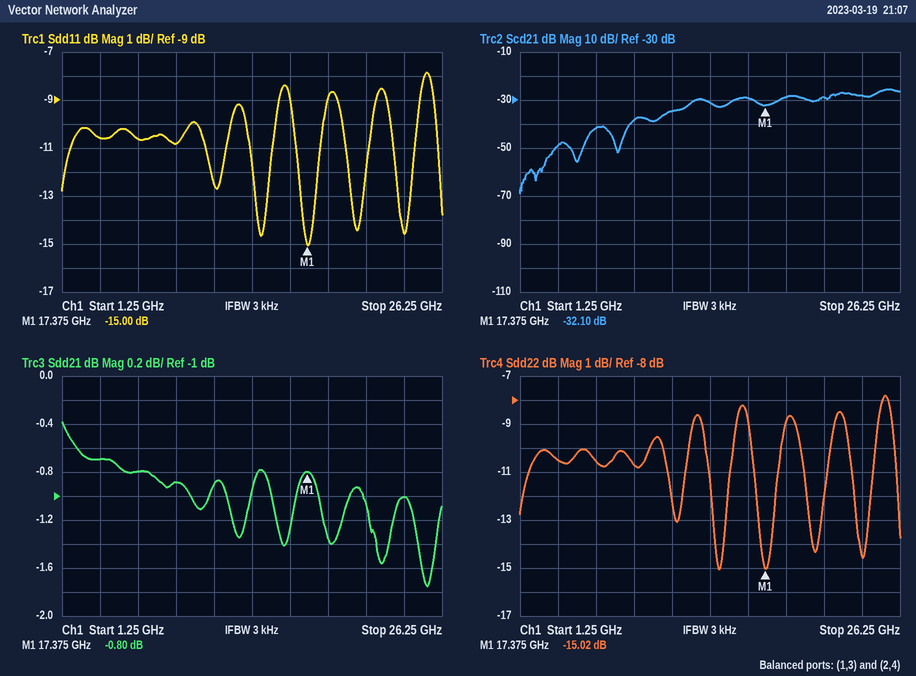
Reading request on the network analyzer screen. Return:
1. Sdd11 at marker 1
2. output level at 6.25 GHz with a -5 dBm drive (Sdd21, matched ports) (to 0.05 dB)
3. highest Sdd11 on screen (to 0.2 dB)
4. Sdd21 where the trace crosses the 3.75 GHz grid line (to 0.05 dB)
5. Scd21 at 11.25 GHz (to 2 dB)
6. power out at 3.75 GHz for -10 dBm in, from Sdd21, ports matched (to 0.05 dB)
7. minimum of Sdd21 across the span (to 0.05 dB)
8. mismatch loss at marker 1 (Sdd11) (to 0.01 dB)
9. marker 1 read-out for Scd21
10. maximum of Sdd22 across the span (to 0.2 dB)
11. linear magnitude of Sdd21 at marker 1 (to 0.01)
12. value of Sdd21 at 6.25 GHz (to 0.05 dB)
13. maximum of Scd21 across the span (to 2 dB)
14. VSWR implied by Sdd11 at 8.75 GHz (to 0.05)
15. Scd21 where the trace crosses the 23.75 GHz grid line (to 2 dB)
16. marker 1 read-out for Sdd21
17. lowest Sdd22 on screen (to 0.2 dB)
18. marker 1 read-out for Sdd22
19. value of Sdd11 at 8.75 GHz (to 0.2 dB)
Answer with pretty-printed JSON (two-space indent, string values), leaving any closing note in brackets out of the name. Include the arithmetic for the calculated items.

{
  "Sdd11 at marker 1": "-15.00 dB",
  "output level at 6.25 GHz with a -5 dBm drive (Sdd21, matched ports)": "-5 dBm + (-0.80 dB) = -5.80 dBm",
  "highest Sdd11 on screen": "-7.8 dB",
  "Sdd21 where the trace crosses the 3.75 GHz grid line": "-0.70 dB",
  "Scd21 at 11.25 GHz": "-34 dB",
  "power out at 3.75 GHz for -10 dBm in, from Sdd21, ports matched": "-10 dBm + (-0.70 dB) = -10.70 dBm",
  "minimum of Sdd21 across the span": "-1.75 dB",
  "mismatch loss at marker 1 (Sdd11)": "−10 log10(1 − 10^(-15/10)) ≈ 0.14 dB",
  "marker 1 read-out for Scd21": "-32.10 dB",
  "maximum of Sdd22 across the span": "-7.8 dB",
  "linear magnitude of Sdd21 at marker 1": "10^(-0.8/20) ≈ 0.91",
  "value of Sdd21 at 6.25 GHz": "-0.80 dB",
  "maximum of Scd21 across the span": "-26 dB",
  "VSWR implied by Sdd11 at 8.75 GHz": "|Γ| = 10^(-10.8/20) = 0.2884; VSWR = (1 + 0.2884)/(1 − 0.2884) ≈ 1.81, so 1.80 to the nearest 0.05",
  "Scd21 where the trace crosses the 23.75 GHz grid line": "-28 dB",
  "marker 1 read-out for Sdd21": "-0.80 dB",
  "lowest Sdd22 on screen": "-15.0 dB",
  "marker 1 read-out for Sdd22": "-15.02 dB",
  "value of Sdd11 at 8.75 GHz": "-10.8 dB"
}
